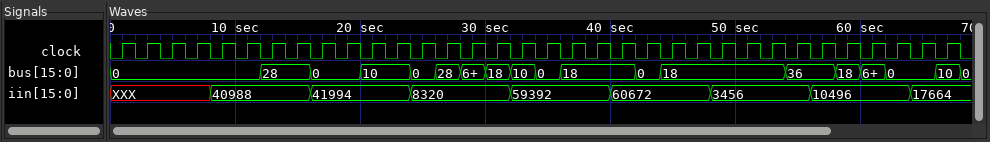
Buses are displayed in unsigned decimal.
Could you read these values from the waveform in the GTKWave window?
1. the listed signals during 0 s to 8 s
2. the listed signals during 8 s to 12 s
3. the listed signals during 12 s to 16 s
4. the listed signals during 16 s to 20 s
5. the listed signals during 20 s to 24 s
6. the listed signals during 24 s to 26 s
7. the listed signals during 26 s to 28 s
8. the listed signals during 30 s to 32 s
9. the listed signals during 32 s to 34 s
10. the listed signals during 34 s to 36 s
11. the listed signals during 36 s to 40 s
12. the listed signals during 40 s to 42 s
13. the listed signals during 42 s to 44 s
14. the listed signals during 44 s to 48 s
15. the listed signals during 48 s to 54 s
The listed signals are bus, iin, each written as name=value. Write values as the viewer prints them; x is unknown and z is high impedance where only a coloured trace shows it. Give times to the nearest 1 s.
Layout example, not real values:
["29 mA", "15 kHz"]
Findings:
["bus=0, iin=XXX", "bus=0, iin=40988", "bus=28, iin=40988", "bus=0, iin=41994", "bus=10, iin=41994", "bus=0, iin=8320", "bus=28, iin=8320", "bus=18, iin=8320", "bus=10, iin=59392", "bus=0, iin=59392", "bus=18, iin=59392", "bus=18, iin=60672", "bus=0, iin=60672", "bus=18, iin=60672", "bus=18, iin=3456"]
